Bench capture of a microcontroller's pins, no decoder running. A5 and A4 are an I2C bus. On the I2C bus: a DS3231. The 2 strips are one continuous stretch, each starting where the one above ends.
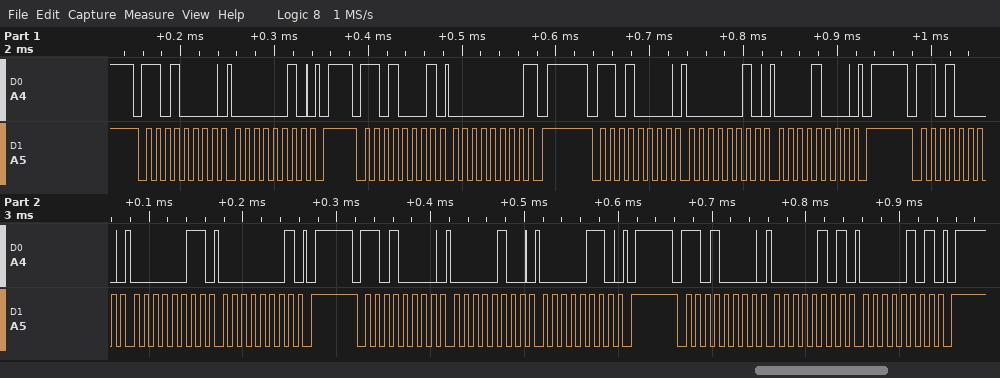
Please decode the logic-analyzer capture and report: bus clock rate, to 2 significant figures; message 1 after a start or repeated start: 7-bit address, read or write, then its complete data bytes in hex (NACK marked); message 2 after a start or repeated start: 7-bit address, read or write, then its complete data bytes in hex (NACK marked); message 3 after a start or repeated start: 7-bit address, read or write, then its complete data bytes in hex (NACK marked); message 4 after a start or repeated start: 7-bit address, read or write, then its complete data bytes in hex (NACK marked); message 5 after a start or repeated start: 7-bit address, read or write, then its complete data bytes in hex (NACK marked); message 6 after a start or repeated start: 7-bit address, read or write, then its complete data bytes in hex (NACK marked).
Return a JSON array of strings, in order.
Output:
["100 kHz", "0x68 write: 02", "0x68 read: 00 NACK", "0x68 write: 02 08", "0x68 write: 03 01", "0x68 write: 04 06", "0x68 write: 05 05"]
